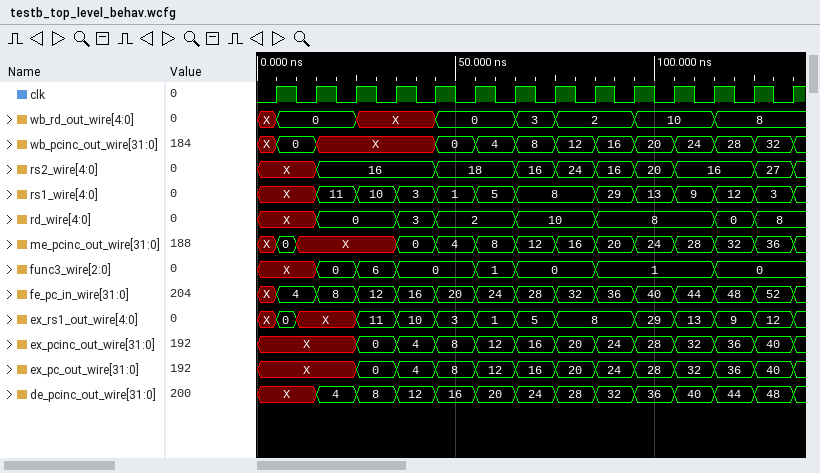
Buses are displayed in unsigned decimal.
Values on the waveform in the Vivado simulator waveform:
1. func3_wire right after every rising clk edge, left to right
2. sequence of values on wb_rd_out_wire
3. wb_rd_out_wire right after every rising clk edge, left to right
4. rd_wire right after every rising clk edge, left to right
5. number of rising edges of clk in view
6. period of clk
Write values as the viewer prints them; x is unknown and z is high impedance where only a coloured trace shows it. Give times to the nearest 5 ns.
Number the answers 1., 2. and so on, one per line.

1. X, 0, 6, 0, 0, 1, 0, 0, 1, 1, 1, 0, 0, 0
2. X, 0, X, 0, 3, 2, 10, 8
3. 0, 0, X, X, 0, 0, 3, 2, 2, 10, 10, 8, 8, 8
4. X, 0, 0, 3, 2, 2, 10, 10, 8, 8, 8, 0, 8, 8
5. 14
6. 10 ns
